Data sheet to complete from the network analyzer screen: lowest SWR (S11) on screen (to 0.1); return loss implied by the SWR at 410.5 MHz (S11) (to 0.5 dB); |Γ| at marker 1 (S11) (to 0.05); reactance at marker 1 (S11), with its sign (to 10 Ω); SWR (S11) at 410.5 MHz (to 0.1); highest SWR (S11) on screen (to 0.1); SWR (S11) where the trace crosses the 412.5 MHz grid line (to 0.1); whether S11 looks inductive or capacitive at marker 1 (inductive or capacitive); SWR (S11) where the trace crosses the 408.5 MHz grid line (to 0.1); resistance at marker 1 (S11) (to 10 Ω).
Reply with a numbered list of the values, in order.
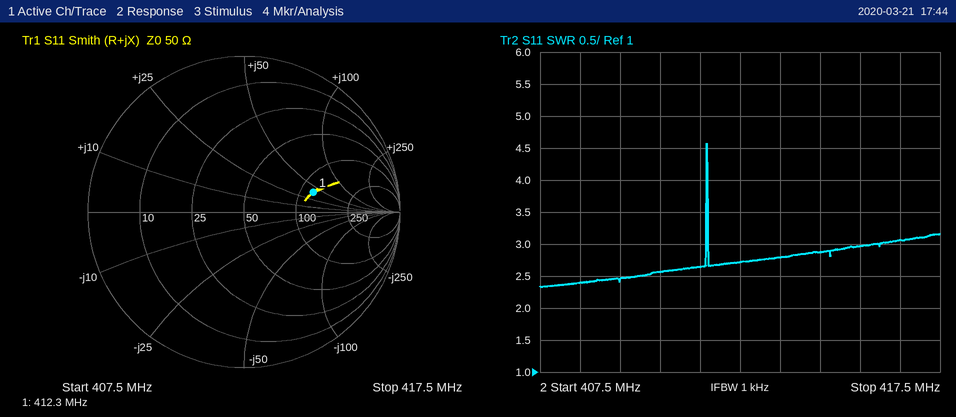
1. 2.3
2. 7.0 dB
3. 0.45
4. +40 Ω
5. 2.6
6. 4.6
7. 2.7
8. inductive
9. 2.4
10. 120 Ω
